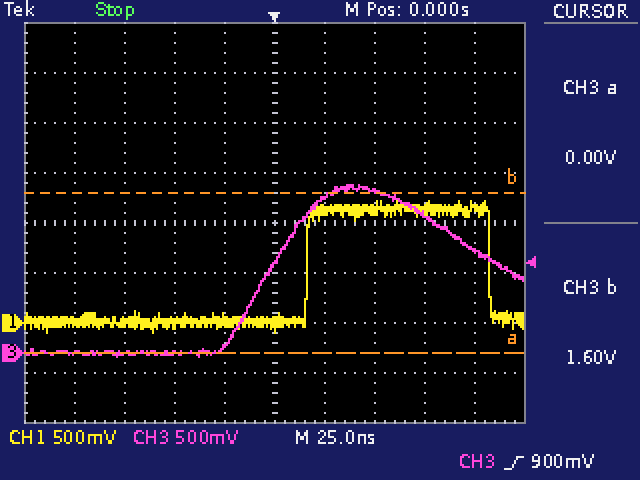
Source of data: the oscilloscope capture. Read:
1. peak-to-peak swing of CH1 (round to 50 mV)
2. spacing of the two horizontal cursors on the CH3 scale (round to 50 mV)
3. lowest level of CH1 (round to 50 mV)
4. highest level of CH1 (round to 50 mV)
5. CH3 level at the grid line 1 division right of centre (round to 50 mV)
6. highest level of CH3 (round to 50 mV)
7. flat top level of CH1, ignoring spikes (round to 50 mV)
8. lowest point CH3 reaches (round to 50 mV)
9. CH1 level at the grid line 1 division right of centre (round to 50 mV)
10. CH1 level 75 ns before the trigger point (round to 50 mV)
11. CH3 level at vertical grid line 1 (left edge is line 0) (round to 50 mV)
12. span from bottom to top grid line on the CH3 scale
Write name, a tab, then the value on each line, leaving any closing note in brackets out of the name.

peak-to-peak swing of CH1	1.30 V
spacing of the two horizontal cursors on the CH3 scale	1.60 V
lowest level of CH1	-100 mV
highest level of CH1	1.20 V
CH3 level at the grid line 1 division right of centre	1.55 V
highest level of CH3	1.70 V
flat top level of CH1, ignoring spikes	1.15 V
lowest point CH3 reaches	-50 mV
CH1 level at the grid line 1 division right of centre	1.15 V
CH1 level 75 ns before the trigger point	0 mV
CH3 level at vertical grid line 1 (left edge is line 0)	0 mV
span from bottom to top grid line on the CH3 scale	4 V
